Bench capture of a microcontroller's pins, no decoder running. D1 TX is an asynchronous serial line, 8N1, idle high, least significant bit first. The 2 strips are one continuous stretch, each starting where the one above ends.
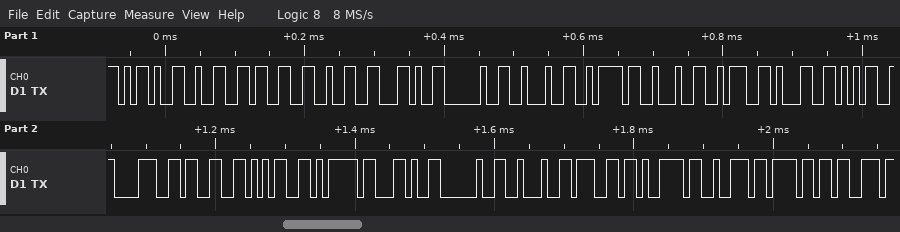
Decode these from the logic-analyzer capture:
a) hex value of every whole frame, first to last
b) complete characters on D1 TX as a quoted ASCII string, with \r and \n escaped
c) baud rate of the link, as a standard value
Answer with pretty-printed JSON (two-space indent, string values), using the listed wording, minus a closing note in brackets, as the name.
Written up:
{
  "hex value of every whole frame, first to last": "2D 32 33 32 2C 20 22 7A 22 3A 31 35 38 33 35 7D 2C 20 22 67 79 72 6F 73",
  "complete characters on D1 TX as a quoted ASCII string, with \\r and \\n escaped": "\"-232, \\\"z\\\":15835}, \\\"gyros\"",
  "baud rate of the link, as a standard value": "115200 baud"
}
